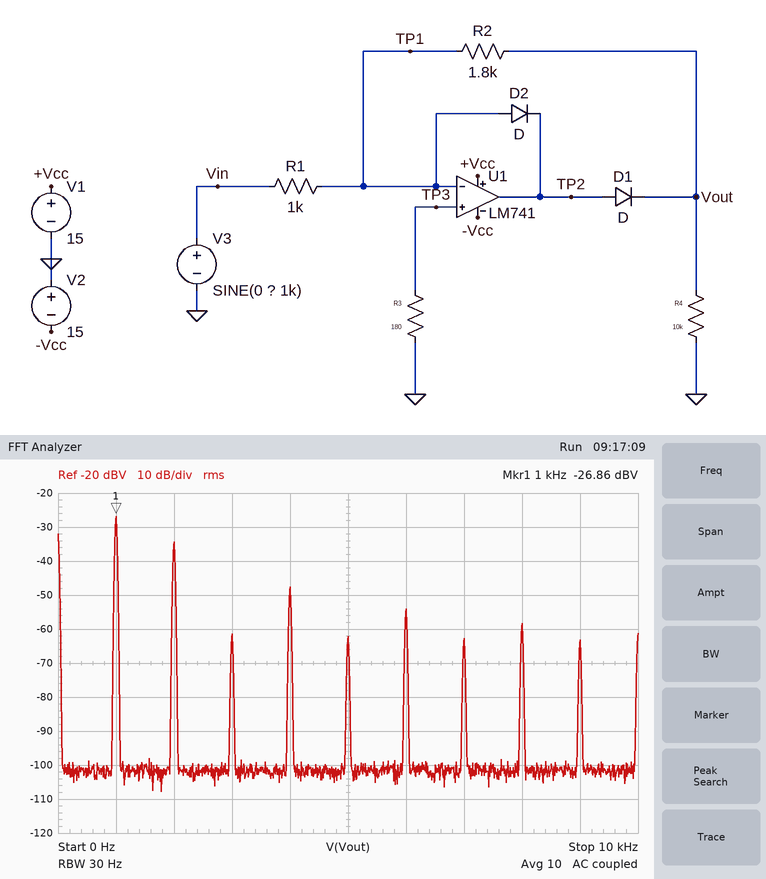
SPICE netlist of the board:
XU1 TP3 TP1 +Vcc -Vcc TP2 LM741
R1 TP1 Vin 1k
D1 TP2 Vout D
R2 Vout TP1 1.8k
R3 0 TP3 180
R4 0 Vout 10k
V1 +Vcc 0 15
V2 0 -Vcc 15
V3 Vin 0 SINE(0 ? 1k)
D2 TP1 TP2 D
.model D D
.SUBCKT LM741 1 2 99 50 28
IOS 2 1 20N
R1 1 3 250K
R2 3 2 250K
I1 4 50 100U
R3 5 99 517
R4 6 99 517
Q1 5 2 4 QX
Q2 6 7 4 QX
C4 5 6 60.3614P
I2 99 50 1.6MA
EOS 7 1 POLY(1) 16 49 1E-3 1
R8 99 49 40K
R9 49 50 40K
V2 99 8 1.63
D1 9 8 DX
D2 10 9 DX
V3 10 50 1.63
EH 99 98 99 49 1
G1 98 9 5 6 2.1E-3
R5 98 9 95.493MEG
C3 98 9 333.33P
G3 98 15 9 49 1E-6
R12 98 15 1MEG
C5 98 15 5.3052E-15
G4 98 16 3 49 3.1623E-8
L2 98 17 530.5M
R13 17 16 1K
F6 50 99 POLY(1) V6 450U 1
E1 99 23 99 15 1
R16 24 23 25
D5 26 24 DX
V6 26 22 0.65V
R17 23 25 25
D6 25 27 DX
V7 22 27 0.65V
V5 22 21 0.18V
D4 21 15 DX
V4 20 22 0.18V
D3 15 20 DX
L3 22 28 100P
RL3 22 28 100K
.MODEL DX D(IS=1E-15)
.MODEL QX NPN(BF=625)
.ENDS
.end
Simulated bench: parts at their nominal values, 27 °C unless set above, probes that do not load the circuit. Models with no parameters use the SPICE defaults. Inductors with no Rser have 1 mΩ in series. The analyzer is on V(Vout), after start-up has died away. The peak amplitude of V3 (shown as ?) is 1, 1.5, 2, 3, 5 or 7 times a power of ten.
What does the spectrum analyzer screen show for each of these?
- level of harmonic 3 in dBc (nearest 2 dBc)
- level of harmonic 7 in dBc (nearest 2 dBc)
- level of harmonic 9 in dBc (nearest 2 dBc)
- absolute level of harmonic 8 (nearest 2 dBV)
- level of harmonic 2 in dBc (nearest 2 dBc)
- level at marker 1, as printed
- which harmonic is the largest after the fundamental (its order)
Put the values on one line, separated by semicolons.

-34 dBc; -36 dBc; -36 dBc; -58 dBV; -8 dBc; -26.86 dBV; 2
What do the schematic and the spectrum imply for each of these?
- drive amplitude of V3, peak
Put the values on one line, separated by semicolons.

70 mV
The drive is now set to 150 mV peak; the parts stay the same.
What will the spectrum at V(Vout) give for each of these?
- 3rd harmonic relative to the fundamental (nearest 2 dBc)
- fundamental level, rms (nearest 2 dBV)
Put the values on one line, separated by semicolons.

-40 dBc; -20 dBV
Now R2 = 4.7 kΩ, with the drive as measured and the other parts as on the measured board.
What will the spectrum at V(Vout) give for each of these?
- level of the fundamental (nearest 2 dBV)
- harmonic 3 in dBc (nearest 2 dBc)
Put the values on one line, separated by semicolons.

-18 dBV; -38 dBc
